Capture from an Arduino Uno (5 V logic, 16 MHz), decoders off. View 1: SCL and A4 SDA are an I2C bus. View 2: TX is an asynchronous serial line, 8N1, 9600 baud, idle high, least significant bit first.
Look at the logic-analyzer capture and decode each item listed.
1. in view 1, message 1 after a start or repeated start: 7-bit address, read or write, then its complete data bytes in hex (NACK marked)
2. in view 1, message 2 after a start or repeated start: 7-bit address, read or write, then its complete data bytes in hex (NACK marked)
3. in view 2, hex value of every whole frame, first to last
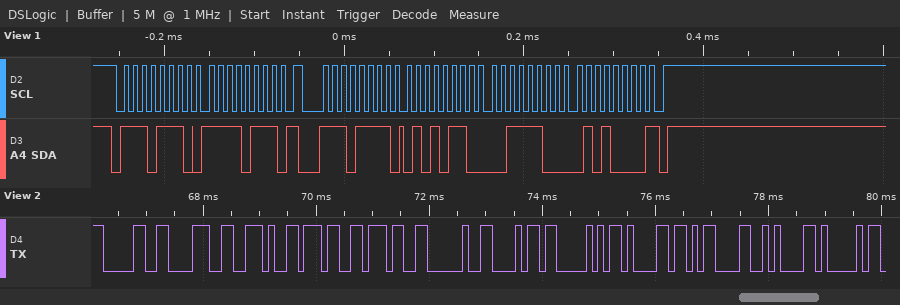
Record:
0x77 write: F7
0x77 read: 56 3C 50 NACK
30 38 2E 37 37 20 68 50 61 0D 0A 41
